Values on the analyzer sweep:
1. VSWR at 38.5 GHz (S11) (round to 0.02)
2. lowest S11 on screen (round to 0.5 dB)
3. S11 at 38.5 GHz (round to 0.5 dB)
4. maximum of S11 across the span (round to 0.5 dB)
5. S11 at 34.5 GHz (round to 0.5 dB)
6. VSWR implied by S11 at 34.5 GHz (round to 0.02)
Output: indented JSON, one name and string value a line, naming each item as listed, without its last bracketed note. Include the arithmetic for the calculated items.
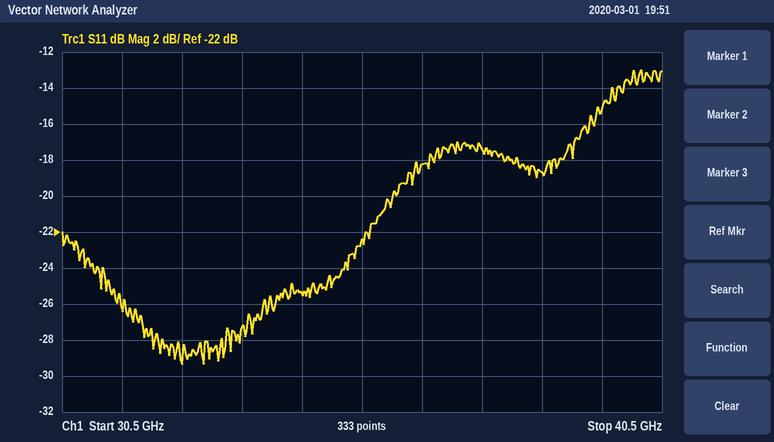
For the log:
{
  "VSWR at 38.5 GHz (S11)": "|Γ| = 10^(-18.5/20) = 0.1189; VSWR = (1 + 0.1189)/(1 − 0.1189) ≈ 1.27, so 1.26 to the nearest 0.02",
  "lowest S11 on screen": "-29.5 dB",
  "S11 at 38.5 GHz": "-18.5 dB",
  "maximum of S11 across the span": "-13.0 dB",
  "S11 at 34.5 GHz": "-25.5 dB",
  "VSWR implied by S11 at 34.5 GHz": "|Γ| = 10^(-25.5/20) = 0.0531; VSWR = (1 + 0.0531)/(1 − 0.0531) ≈ 1.11, so 1.12 to the nearest 0.02"
}
